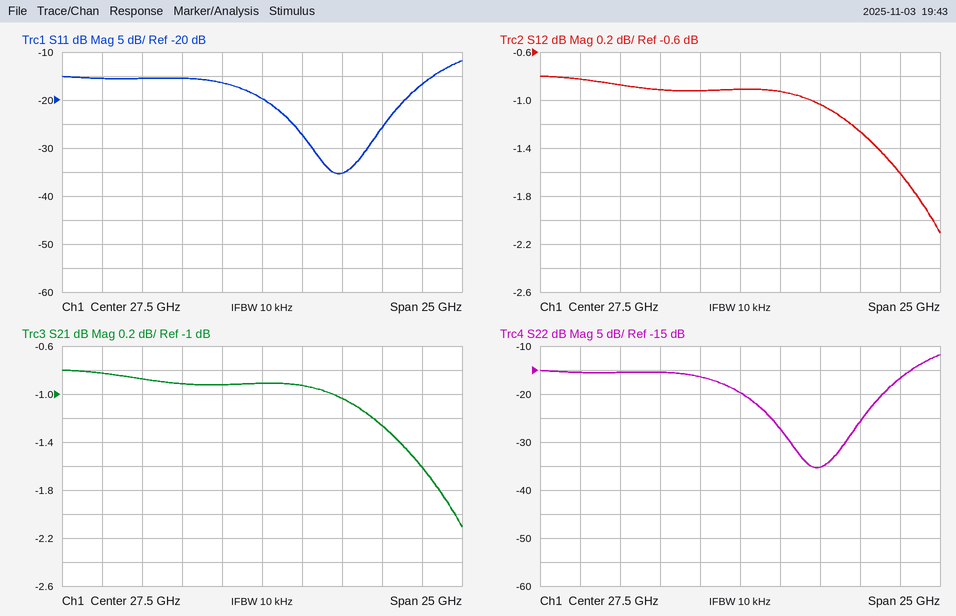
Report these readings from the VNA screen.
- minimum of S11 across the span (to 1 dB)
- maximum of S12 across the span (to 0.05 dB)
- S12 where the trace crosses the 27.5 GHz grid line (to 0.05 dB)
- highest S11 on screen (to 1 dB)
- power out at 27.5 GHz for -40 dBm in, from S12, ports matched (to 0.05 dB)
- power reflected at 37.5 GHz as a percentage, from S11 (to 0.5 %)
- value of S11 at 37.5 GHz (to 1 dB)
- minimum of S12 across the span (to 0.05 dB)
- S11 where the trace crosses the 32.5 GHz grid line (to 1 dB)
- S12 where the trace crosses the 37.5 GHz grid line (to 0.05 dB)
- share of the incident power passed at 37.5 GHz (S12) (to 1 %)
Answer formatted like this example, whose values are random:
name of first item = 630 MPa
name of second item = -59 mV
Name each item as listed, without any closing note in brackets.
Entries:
minimum of S11 across the span = -35 dB
maximum of S12 across the span = -0.80 dB
S12 where the trace crosses the 27.5 GHz grid line = -0.90 dB
highest S11 on screen = -12 dB
power out at 27.5 GHz for -40 dBm in, from S12, ports matched = -40.90 dBm
power reflected at 37.5 GHz as a percentage, from S11 = 2.0 %
value of S11 at 37.5 GHz = -17 dB
minimum of S12 across the span = -2.10 dB
S11 where the trace crosses the 32.5 GHz grid line = -35 dB
S12 where the trace crosses the 37.5 GHz grid line = -1.60 dB
share of the incident power passed at 37.5 GHz (S12) = 69 %
